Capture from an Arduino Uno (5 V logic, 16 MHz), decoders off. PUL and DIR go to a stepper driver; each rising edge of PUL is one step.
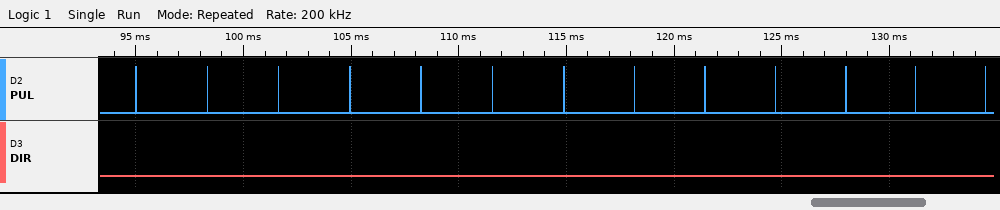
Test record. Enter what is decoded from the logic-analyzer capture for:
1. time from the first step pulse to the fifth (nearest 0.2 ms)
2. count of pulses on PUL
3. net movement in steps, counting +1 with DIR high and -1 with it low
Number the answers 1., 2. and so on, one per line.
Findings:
1. 13.2 ms
2. 13
3. -13
